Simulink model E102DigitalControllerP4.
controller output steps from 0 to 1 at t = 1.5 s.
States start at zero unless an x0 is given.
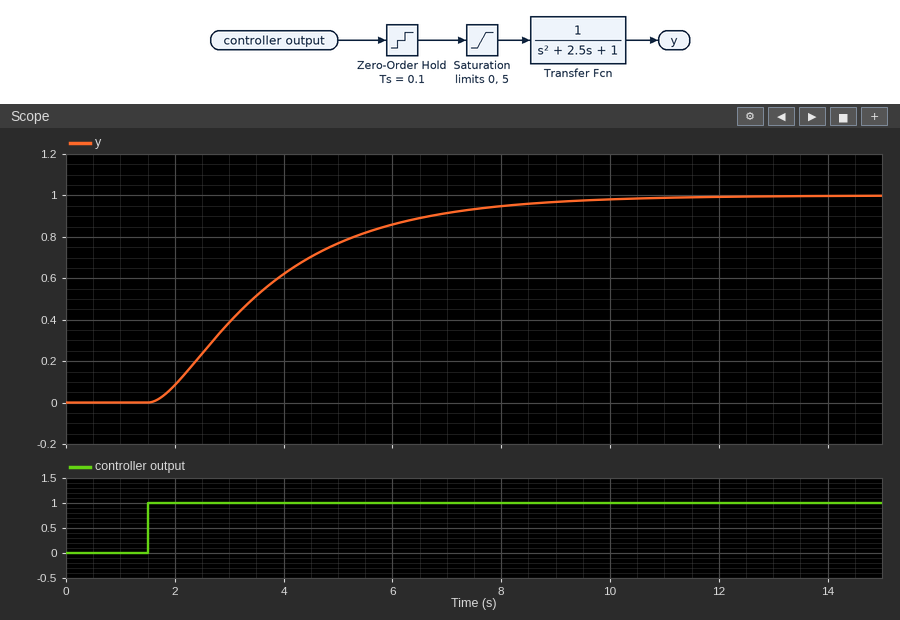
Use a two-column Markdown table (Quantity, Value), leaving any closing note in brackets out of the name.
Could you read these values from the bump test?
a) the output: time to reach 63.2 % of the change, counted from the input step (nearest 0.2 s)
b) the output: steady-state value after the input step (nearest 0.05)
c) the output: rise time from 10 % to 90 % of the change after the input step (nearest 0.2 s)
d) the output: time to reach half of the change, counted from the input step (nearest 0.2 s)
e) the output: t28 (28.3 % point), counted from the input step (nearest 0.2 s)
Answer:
| Quantity | Value |
|---|---|
| the output: time to reach 63.2 % of the change, counted from the input step | 2.6 s |
| the output: steady-state value after the input step | 1.00 |
| the output: rise time from 10 % to 90 % of the change after the input step | 4.6 s |
| the output: time to reach half of the change, counted from the input step | 2.0 s |
| the output: t28 (28.3 % point), counted from the input step | 1.2 s |
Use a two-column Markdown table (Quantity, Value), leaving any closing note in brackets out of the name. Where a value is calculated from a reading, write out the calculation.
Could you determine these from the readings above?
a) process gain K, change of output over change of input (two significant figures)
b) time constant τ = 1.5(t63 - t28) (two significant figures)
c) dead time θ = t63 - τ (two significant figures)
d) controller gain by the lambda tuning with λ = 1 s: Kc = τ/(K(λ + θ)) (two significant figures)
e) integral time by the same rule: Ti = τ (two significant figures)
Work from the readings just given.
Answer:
| Quantity | Value |
|---|---|
| process gain K, change of output over change of input | (1 - 0) / 1 = 1.0 |
| time constant τ = 1.5(t63 - t28) | 1.5 × (2.6 - 1.2) = 2.1 s |
| dead time θ = t63 - τ | 2.6 - 2.1 = 0.50 s |
| controller gain by the lambda tuning with λ = 1 s: Kc = τ/(K(λ + θ)) | 2.1 / (1 × (1 + 0.5)) = 1.4 |
| integral time by the same rule: Ti = τ | 2.1 s |
